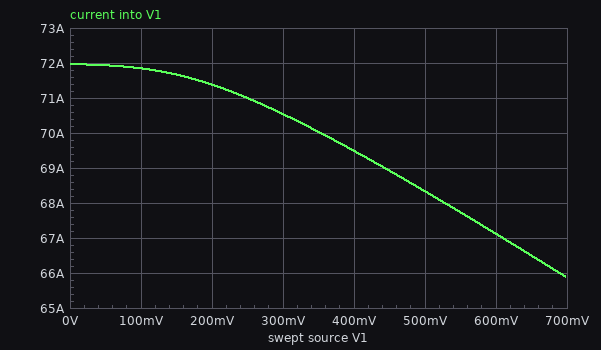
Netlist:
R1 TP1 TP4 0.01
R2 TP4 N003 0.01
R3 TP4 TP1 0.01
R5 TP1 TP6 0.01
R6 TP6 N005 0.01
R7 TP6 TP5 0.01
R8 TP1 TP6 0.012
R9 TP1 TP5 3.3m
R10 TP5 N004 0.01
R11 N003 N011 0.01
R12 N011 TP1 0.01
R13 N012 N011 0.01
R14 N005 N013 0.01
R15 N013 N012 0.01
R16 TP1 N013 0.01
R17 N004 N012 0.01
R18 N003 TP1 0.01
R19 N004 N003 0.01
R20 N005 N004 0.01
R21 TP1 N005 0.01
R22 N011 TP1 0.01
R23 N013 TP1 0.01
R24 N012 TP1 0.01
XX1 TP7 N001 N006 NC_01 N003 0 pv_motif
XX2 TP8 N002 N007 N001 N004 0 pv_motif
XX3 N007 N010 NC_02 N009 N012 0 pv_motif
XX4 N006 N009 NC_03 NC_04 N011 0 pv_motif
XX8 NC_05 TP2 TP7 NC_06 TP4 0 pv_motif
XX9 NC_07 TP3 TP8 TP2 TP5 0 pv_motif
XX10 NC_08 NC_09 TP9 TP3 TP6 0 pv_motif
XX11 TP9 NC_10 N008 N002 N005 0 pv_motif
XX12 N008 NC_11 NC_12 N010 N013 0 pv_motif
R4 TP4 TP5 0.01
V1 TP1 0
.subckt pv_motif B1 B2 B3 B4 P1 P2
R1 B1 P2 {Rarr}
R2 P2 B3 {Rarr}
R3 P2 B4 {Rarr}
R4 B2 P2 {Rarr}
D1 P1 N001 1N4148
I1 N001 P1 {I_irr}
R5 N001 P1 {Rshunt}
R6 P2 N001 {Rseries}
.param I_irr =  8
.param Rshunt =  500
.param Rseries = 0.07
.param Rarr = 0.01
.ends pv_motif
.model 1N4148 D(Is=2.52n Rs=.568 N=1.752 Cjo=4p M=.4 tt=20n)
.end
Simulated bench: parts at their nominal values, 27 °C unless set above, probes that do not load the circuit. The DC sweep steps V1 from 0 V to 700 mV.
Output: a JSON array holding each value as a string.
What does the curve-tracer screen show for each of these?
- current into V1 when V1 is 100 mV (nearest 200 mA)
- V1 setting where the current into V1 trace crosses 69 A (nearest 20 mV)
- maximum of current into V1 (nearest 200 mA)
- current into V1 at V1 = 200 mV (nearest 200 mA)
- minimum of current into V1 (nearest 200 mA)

["71.8 A", "440 mV", "72.0 A", "71.4 A", "65.8 A"]
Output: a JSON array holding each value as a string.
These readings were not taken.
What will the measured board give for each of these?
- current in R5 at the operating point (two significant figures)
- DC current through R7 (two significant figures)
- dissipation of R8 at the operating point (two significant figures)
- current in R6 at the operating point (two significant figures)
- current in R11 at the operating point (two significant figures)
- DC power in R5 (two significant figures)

["4.9 A", "660 mA", "200 mW", "1.6 A", "1.2 A", "240 mW"]
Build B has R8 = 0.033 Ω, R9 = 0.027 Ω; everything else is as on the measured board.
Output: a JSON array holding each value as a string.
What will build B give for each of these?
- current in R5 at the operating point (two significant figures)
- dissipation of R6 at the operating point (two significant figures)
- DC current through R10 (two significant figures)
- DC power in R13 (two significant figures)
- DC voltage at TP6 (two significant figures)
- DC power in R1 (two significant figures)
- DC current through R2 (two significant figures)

["7.7 A", "440 µW", "580 mA", "28 mW", "77 mV", "390 mW", "1.3 A"]
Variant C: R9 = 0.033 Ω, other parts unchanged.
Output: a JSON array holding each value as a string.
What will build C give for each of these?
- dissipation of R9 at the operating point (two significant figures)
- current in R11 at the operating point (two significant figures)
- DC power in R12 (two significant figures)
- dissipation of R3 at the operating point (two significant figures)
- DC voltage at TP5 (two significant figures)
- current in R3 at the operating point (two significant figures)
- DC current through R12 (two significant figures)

["260 mW", "1.7 A", "320 mW", "380 mW", "92 mV", "6.2 A", "5.7 A"]
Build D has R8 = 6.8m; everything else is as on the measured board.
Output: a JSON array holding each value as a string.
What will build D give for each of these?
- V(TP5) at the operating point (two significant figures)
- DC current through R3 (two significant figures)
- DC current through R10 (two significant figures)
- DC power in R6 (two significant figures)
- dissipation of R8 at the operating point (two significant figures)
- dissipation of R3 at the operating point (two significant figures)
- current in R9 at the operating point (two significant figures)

["41 mV", "4.6 A", "3.8 A", "48 mW", "250 mW", "210 mW", "12 A"]
